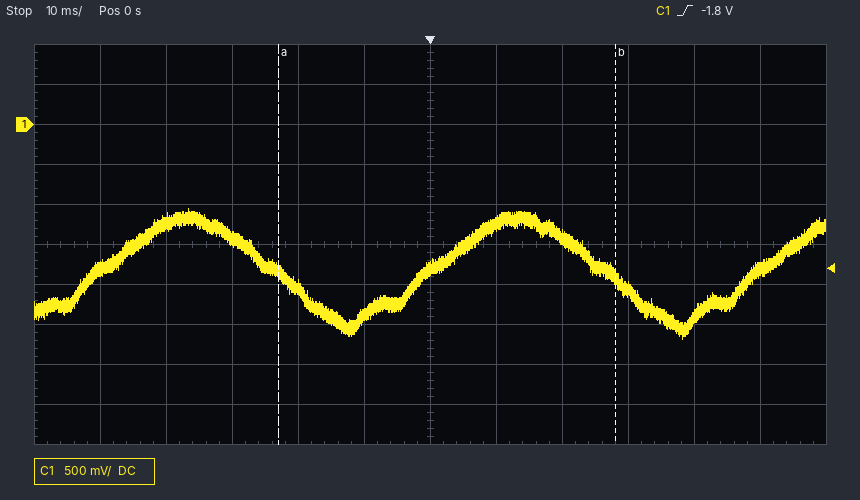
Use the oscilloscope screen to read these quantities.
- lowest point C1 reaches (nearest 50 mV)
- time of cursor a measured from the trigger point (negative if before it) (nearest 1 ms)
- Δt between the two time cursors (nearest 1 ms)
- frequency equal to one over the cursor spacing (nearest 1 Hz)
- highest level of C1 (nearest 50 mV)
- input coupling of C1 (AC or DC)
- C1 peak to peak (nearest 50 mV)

-2.70 V
-23 ms
51 ms
20 Hz
-1.05 V
DC
1.65 V
